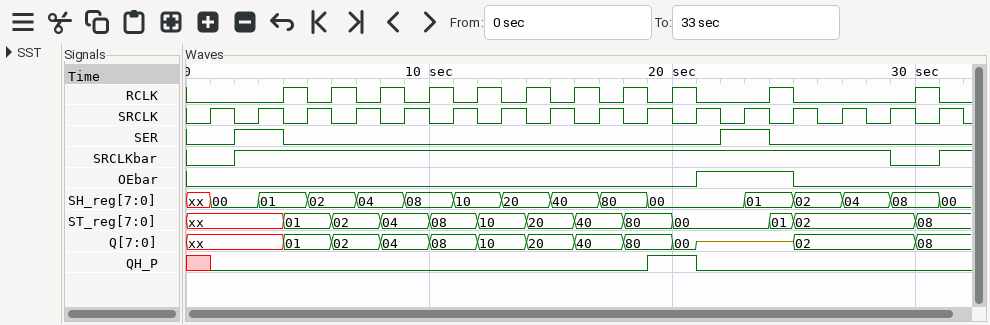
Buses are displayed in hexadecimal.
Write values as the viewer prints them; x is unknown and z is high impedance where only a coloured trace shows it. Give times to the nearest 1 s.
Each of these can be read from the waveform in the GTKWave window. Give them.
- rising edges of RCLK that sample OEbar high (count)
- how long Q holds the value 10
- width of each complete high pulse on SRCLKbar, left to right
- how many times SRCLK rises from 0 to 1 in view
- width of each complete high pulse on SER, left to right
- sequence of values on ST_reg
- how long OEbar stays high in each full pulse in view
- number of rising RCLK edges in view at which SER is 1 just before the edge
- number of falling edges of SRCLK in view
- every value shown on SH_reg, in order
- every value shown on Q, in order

1
2 s
27 s
16
2 s, 2 s
xx, 01, 02, 04, 08, 10, 20, 40, 80, 00, 01, 02, 08
4 s
2
16
xx, 00, 01, 02, 04, 08, 10, 20, 40, 80, 00, 01, 02, 04, 08, 00
xx, 01, 02, 04, 08, 10, 20, 40, 80, 00, z, 02, 08
